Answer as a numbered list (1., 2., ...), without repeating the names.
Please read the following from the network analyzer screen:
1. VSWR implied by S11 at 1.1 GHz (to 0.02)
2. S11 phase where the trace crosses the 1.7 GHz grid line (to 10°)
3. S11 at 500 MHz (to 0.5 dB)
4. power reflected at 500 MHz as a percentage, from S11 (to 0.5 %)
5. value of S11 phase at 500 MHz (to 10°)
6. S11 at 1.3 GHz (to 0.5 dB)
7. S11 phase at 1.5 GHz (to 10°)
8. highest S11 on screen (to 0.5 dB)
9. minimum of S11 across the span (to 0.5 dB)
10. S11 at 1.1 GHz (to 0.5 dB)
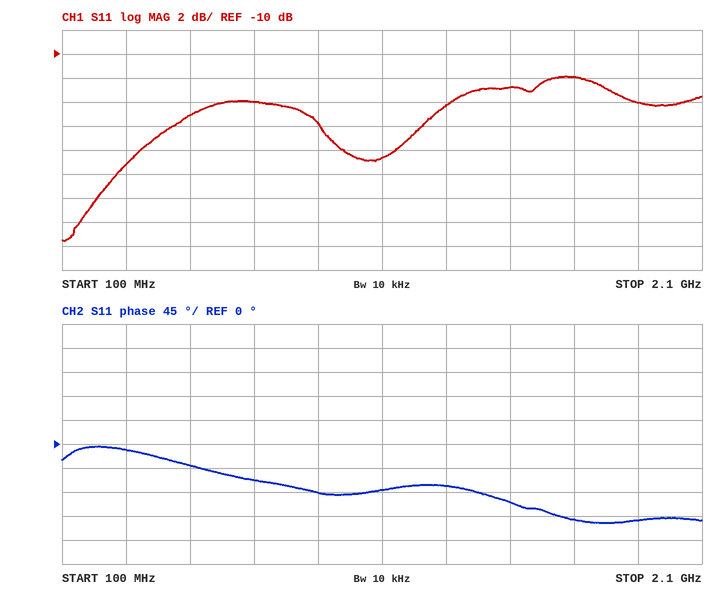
1. 1.26
2. -140°
3. -15.0 dB
4. 3.0 %
5. -40°
6. -14.5 dB
7. -110°
8. -12.0 dB
9. -25.5 dB
10. -18.5 dB
